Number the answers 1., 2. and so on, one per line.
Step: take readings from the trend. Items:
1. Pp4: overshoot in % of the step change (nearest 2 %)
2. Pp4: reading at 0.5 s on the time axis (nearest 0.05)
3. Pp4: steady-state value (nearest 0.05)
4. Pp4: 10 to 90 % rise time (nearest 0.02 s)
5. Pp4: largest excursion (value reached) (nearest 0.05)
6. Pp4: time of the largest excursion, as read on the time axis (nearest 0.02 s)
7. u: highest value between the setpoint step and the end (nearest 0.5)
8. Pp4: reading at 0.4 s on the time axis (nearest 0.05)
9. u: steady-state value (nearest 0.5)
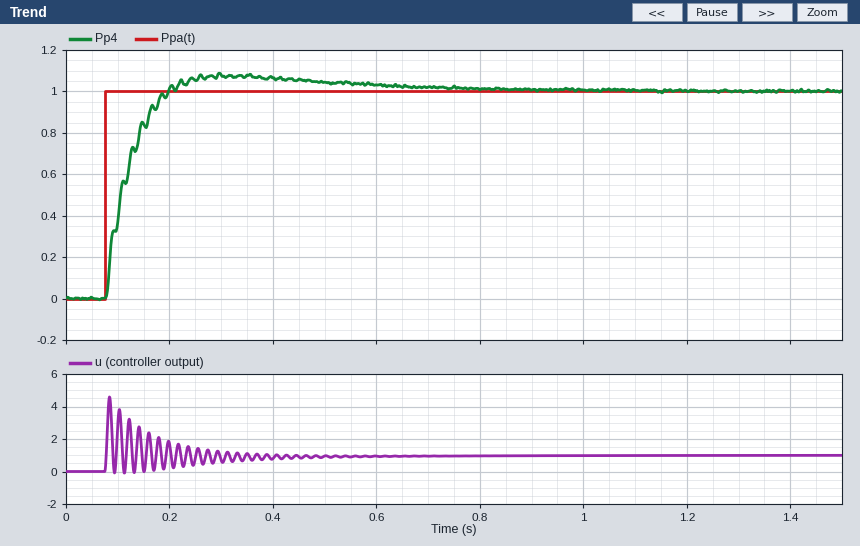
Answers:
1. 8 %
2. 1.05
3. 1.00
4. 0.08 s
5. 1.10
6. 0.30 s
7. 4.5
8. 1.05
9. 1.0
